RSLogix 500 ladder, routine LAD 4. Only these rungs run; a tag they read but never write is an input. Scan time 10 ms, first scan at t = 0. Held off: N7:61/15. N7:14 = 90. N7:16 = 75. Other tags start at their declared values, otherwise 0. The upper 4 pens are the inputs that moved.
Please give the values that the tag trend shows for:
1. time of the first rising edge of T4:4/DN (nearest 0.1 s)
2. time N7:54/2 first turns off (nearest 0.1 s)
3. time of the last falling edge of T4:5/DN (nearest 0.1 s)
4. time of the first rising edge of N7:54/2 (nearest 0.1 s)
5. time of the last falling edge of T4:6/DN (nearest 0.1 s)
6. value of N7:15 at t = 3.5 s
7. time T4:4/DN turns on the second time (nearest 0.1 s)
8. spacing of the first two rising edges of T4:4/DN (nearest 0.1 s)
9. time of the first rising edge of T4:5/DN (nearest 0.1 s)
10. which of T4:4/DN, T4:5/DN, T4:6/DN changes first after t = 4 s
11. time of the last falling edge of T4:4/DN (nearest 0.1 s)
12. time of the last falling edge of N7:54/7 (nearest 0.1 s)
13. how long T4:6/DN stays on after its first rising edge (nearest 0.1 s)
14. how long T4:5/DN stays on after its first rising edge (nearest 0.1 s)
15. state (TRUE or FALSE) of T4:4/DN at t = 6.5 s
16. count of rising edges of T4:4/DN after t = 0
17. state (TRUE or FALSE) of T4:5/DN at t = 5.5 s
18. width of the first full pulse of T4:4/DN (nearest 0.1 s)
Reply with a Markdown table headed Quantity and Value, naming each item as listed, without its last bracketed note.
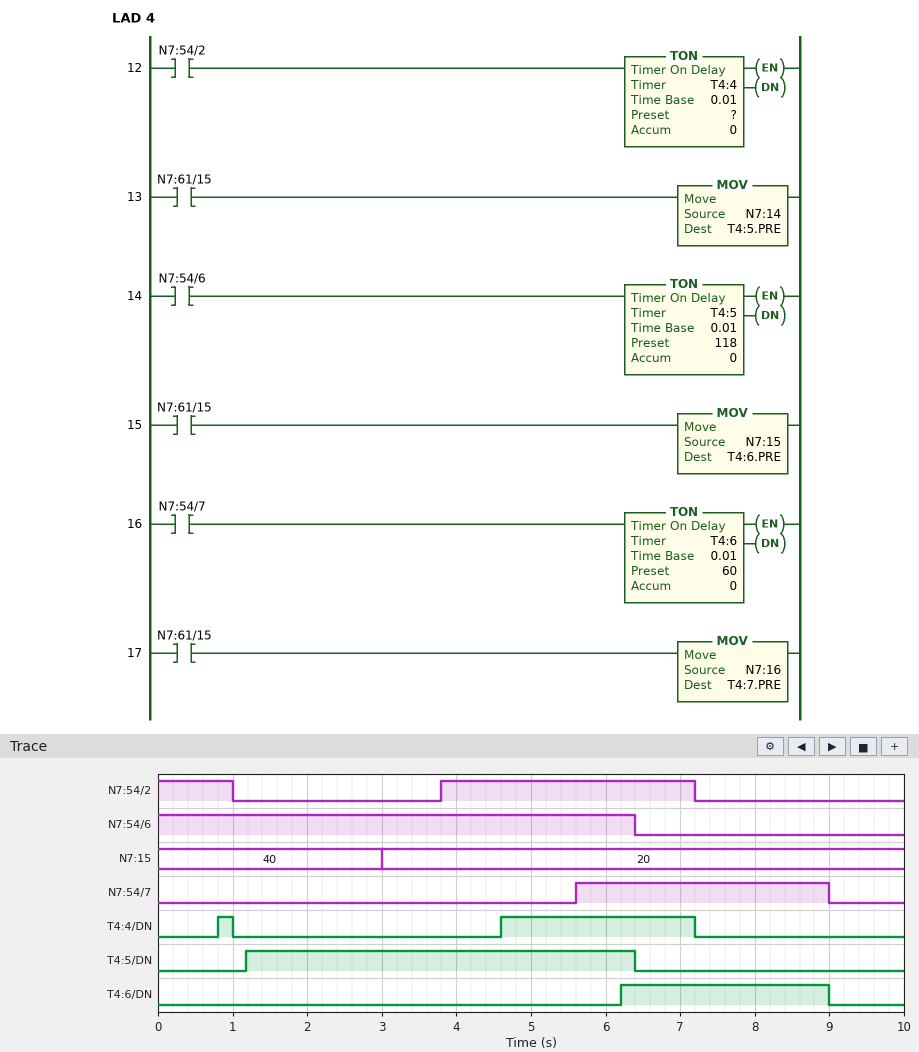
| Quantity | Value |
|---|---|
| time of the first rising edge of T4:4/DN | 0.8 s |
| time N7:54/2 first turns off | 1.0 s |
| time of the last falling edge of T4:5/DN | 6.4 s |
| time of the first rising edge of N7:54/2 | 3.8 s |
| time of the last falling edge of T4:6/DN | 9.0 s |
| value of N7:15 at t = 3.5 s | 20 |
| time T4:4/DN turns on the second time | 4.6 s |
| spacing of the first two rising edges of T4:4/DN | 3.8 s |
| time of the first rising edge of T4:5/DN | 1.2 s |
| which of T4:4/DN, T4:5/DN, T4:6/DN changes first after t = 4 s | T4:4/DN |
| time of the last falling edge of T4:4/DN | 7.2 s |
| time of the last falling edge of N7:54/7 | 9.0 s |
| how long T4:6/DN stays on after its first rising edge | 2.8 s |
| how long T4:5/DN stays on after its first rising edge | 5.2 s |
| state (TRUE or FALSE) of T4:4/DN at t = 6.5 s | TRUE |
| count of rising edges of T4:4/DN after t = 0 | 2 |
| state (TRUE or FALSE) of T4:5/DN at t = 5.5 s | TRUE |
| width of the first full pulse of T4:4/DN | 0.2 s |
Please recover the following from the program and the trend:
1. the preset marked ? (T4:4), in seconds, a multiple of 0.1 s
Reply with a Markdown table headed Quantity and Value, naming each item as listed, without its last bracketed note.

| Quantity | Value |
|---|---|
| the preset marked ? (T4:4), in seconds, a multiple of 0.1 s | 0.8 s |
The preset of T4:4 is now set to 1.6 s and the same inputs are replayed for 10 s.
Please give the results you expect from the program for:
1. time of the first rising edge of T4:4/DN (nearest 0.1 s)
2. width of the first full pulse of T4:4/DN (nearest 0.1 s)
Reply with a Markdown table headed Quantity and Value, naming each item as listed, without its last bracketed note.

| Quantity | Value |
|---|---|
| time of the first rising edge of T4:4/DN | 5.4 s |
| width of the first full pulse of T4:4/DN | 1.8 s |
